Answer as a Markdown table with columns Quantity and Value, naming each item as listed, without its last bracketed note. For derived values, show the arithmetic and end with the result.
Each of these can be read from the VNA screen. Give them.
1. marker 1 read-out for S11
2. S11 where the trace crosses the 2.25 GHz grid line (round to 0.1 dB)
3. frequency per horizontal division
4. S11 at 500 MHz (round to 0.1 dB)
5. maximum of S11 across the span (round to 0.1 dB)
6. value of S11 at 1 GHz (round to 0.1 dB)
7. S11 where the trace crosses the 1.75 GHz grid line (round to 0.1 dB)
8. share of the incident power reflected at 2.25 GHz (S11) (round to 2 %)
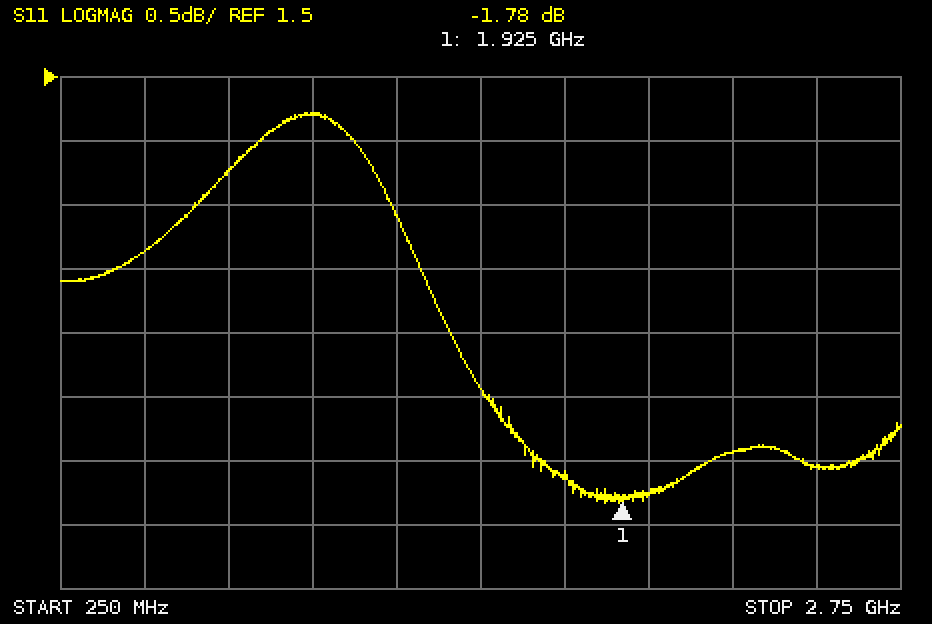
| Quantity | Value |
|---|---|
| marker 1 read-out for S11 | -1.78 dB |
| S11 where the trace crosses the 2.25 GHz grid line | -1.4 dB |
| frequency per horizontal division | 250 MHz |
| S11 at 500 MHz | 0.1 dB |
| maximum of S11 across the span | 1.2 dB |
| value of S11 at 1 GHz | 1.2 dB |
| S11 where the trace crosses the 1.75 GHz grid line | -1.6 dB |
| share of the incident power reflected at 2.25 GHz (S11) | 10^(-1.4/10) ≈ 72 % |
